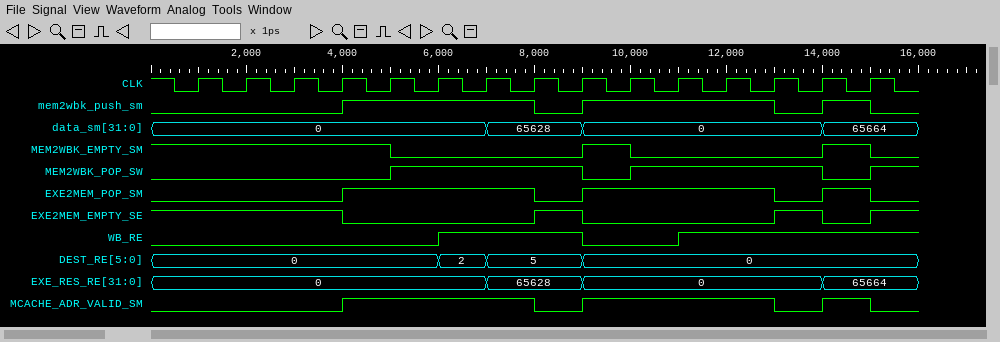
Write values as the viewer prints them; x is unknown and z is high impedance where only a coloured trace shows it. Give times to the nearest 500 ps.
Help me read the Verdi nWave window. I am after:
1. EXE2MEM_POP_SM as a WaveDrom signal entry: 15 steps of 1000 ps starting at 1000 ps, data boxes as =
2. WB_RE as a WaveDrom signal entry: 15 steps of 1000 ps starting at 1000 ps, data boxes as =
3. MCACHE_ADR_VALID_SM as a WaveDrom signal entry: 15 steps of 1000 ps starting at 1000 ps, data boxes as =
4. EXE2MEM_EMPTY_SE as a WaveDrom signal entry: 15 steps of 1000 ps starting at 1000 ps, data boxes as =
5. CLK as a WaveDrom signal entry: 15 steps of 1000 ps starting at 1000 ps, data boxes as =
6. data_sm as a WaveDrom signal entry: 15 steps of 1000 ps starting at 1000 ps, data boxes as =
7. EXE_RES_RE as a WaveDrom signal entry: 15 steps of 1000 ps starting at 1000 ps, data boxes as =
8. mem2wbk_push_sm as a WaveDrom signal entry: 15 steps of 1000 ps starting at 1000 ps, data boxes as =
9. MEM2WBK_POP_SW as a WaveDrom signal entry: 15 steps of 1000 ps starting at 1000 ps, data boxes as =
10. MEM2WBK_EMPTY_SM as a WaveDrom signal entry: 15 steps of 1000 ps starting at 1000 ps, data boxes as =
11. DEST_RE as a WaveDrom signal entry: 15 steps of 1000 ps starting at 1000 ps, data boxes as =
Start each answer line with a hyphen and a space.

- {name: 'EXE2MEM_POP_SM', wave: '0..1...01...010'}
- {name: 'WB_RE', wave: '0....1..0.1....'}
- {name: 'MCACHE_ADR_VALID_SM', wave: '0..1...01...010'}
- {name: 'EXE2MEM_EMPTY_SE', wave: '1..0...10...101'}
- {name: 'CLK', wave: 'p..............'}
- {name: 'data_sm', wave: '=.....=.=....=.', data: '0 65628 0 65664'}
- {name: 'EXE_RES_RE', wave: '=.....=.=....=.', data: '0 65628 0 65664'}
- {name: 'mem2wbk_push_sm', wave: '0..1...01...010'}
- {name: 'MEM2WBK_POP_SW', wave: '0...1...01...01'}
- {name: 'MEM2WBK_EMPTY_SM', wave: '1...0...10...10'}
- {name: 'DEST_RE', wave: '=....==.=......', data: '0 2 5 0'}
